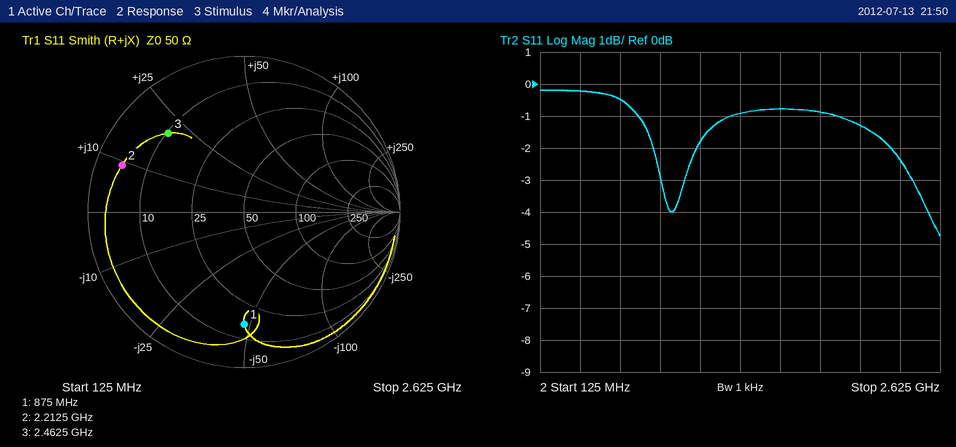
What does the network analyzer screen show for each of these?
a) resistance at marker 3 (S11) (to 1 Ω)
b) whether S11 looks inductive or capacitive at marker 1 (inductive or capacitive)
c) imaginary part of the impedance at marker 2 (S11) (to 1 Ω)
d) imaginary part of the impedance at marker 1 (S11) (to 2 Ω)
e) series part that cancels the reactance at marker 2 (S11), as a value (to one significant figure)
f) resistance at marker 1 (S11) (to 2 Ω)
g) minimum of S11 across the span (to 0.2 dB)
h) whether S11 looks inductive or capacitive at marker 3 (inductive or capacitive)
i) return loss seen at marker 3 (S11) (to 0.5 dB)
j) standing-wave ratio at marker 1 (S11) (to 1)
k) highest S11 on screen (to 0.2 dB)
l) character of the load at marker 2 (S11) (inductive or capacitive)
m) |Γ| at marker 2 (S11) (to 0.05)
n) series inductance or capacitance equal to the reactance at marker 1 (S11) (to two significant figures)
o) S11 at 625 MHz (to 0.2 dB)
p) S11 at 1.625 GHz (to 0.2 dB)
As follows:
10 Ω
capacitive
+9 Ω
-48 Ω
8 pF
16 Ω
-4.8 dB
inductive
3.0 dB
6
-0.2 dB
inductive
0.85
3.8 pF
-0.4 dB
-0.8 dB
